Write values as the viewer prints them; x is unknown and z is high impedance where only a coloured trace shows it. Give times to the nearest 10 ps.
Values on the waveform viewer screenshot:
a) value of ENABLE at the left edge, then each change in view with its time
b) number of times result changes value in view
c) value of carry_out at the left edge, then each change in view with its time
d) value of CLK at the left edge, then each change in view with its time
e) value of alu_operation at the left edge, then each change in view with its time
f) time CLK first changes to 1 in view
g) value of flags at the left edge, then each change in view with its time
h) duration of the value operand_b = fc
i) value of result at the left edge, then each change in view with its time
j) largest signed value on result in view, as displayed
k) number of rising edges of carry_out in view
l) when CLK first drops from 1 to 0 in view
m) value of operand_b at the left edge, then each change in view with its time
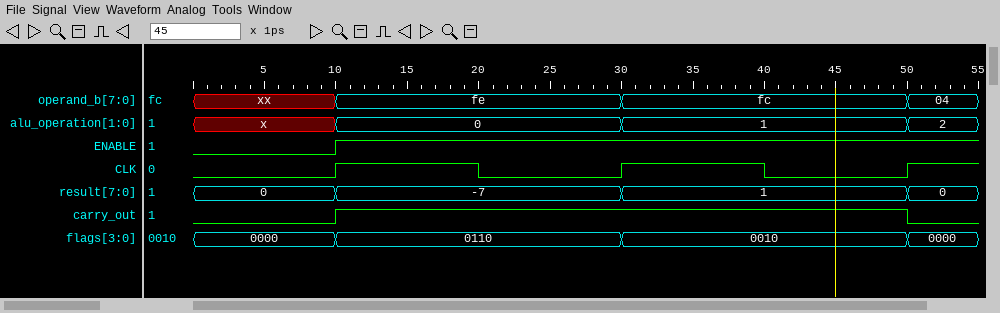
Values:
0, 1 at 10 ps
3
0, 1 at 10 ps, 0 at 50 ps
0, 1 at 10 ps, 0 at 20 ps, 1 at 30 ps, 0 at 40 ps, 1 at 50 ps
x, 0 at 10 ps, 1 at 30 ps, 2 at 50 ps
10 ps
0000, 0110 at 10 ps, 0010 at 30 ps, 0000 at 50 ps
20 ps
0, -7 at 10 ps, 1 at 30 ps, 0 at 50 ps
1
1
20 ps
xx, fe at 10 ps, fc at 30 ps, 04 at 50 ps
